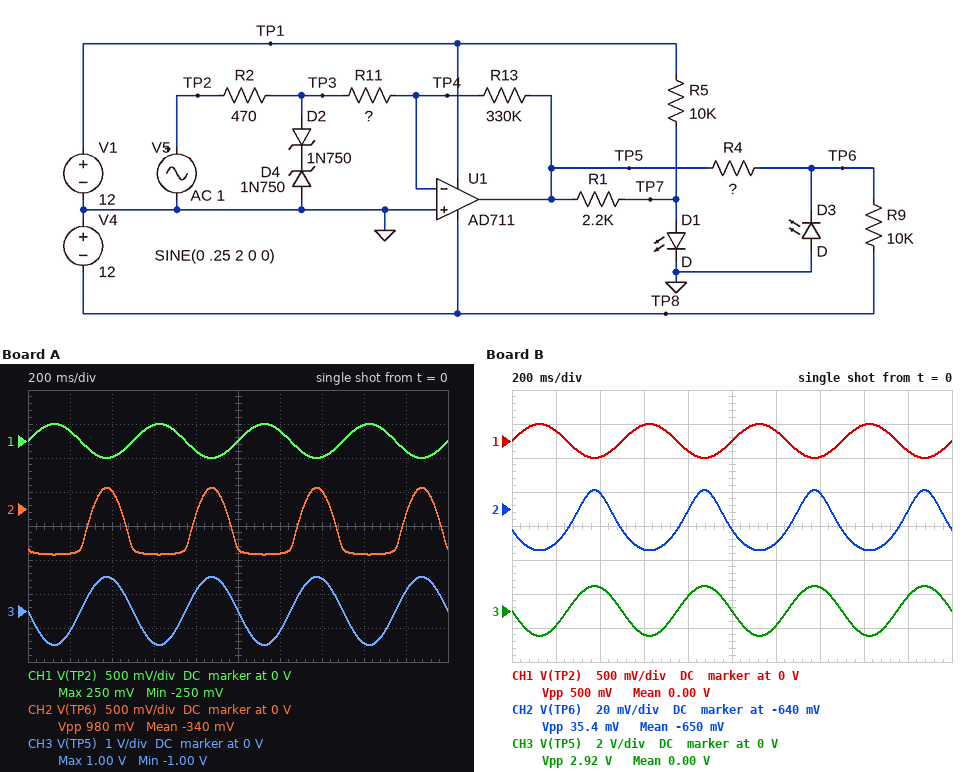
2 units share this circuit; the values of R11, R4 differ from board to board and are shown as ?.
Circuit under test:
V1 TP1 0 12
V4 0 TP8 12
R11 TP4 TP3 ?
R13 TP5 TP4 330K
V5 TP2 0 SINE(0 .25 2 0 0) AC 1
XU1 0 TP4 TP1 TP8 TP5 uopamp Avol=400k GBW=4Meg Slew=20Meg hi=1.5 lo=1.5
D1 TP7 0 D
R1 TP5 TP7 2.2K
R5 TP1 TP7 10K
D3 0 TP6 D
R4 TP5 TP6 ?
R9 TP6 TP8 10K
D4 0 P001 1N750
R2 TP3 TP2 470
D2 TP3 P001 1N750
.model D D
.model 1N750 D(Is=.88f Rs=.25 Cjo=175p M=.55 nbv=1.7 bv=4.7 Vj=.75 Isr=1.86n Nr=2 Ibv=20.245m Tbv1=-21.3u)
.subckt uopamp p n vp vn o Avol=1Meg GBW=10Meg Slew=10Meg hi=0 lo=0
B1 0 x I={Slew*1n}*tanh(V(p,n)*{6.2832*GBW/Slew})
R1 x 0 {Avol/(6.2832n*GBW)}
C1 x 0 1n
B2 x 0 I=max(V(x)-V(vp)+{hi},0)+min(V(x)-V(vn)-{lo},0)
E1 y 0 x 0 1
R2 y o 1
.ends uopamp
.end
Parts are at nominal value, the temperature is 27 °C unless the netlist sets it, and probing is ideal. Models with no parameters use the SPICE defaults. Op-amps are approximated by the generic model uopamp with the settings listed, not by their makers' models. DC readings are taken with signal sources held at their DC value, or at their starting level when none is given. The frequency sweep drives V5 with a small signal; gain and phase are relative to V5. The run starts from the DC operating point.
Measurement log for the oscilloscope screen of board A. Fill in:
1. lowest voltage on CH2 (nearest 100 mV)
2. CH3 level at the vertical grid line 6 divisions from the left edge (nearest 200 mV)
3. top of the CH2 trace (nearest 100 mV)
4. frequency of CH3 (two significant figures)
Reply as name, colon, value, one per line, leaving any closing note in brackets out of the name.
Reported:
lowest voltage on CH2: -700 mV
CH3 level at the vertical grid line 6 divisions from the left edge: -600 mV
top of the CH2 trace: 300 mV
frequency of CH3: 2.0 Hz
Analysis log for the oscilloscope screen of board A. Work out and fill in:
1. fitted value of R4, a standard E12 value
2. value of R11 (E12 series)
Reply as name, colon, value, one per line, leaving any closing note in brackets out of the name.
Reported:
fitted value of R4, a standard E12 value: 560 Ω
value of R11: 82 kΩ
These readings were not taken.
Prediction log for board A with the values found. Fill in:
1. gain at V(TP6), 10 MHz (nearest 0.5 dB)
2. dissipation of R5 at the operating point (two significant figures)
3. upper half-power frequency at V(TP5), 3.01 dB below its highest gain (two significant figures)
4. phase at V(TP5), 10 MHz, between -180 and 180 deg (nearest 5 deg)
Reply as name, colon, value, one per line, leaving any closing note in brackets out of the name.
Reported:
gain at V(TP6), 10 MHz: -28.0 dB
dissipation of R5 at the operating point: 13 mW
upper half-power frequency at V(TP5), 3.01 dB below its highest gain: 770 kHz
phase at V(TP5), 10 MHz, between -180 and 180 deg: 25 deg
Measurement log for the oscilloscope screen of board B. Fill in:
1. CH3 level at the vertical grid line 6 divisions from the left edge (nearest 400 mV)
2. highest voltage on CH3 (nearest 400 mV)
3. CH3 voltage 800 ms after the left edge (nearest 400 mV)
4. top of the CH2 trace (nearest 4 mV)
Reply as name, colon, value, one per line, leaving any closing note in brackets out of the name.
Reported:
CH3 level at the vertical grid line 6 divisions from the left edge: -800 mV
highest voltage on CH3: 1.6 V
CH3 voltage 800 ms after the left edge: 800 mV
top of the CH2 trace: -628 mV
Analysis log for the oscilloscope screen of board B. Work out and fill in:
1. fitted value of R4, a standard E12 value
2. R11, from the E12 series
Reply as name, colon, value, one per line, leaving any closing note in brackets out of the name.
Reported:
fitted value of R4, a standard E12 value: 2.7 kΩ
R11, from the E12 series: 56 kΩ
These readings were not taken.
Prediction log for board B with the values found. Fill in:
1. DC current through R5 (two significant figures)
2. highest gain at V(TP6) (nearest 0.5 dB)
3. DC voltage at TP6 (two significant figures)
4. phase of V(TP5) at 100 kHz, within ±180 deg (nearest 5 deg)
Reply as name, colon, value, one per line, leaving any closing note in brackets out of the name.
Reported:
DC current through R5: 1.1 mA
highest gain at V(TP6): -24.0 dB
DC voltage at TP6: -650 mV
phase of V(TP5) at 100 kHz, within ±180 deg: 170 deg
